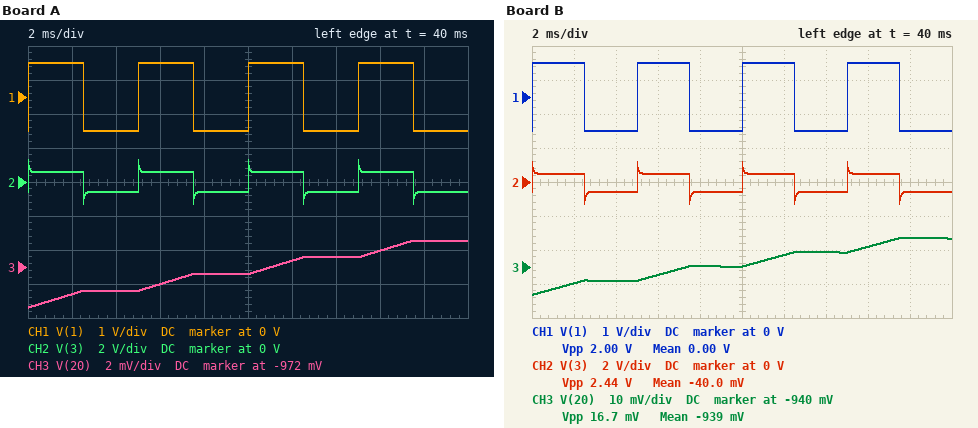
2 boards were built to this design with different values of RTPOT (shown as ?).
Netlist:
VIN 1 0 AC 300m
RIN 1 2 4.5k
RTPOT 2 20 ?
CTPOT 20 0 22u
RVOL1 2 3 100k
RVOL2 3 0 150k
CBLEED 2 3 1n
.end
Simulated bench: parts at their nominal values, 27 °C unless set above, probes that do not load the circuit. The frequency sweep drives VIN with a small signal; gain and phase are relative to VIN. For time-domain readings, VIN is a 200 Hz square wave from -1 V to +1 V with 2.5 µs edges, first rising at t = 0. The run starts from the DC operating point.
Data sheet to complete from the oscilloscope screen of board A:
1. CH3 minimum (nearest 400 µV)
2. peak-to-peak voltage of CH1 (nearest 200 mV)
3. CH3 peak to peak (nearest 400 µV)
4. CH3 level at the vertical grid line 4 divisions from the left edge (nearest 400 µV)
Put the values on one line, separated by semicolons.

-974.4 mV; 2.0 V; 4.0 mV; -972.4 mV
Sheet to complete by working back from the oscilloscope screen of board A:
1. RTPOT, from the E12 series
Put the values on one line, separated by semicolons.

220 kΩ
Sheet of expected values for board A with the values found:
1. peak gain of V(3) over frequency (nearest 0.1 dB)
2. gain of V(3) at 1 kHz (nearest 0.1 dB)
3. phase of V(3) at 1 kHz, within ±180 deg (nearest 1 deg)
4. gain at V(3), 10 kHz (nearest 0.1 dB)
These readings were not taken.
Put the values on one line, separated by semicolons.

-0.4 dB; -3.9 dB; 11 deg; -0.6 dB
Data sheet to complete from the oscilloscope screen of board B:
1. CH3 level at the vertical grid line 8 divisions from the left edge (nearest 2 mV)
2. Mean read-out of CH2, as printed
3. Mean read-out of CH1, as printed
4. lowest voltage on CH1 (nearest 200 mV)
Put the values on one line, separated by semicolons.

-934 mV; -40.0 mV; 0.00 V; -1.0 V
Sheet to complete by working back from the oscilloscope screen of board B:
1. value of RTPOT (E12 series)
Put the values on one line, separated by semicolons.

47 kΩ
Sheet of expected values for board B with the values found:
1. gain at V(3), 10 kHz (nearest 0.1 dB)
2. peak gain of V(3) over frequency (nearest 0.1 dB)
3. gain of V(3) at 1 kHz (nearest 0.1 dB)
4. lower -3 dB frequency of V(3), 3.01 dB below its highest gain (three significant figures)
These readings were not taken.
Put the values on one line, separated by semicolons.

-1.2 dB; -1.0 dB; -4.5 dB; 1.35 kHz
